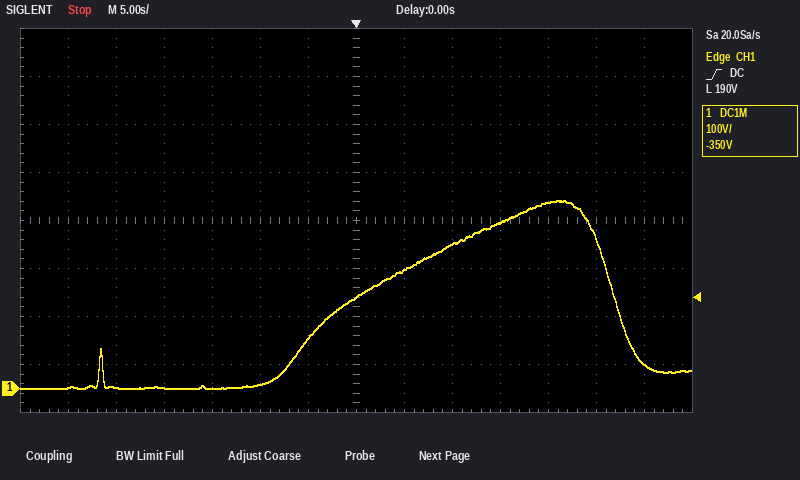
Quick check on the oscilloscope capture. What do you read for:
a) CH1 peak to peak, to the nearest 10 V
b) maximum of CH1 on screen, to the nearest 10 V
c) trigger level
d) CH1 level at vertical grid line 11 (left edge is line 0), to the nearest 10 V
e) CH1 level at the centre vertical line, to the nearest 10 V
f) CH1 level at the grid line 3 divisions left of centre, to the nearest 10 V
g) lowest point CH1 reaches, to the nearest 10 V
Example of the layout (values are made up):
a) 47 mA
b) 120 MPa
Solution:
a) 390 V
b) 390 V
c) 190 V
d) 390 V
e) 190 V
f) 0 V
g) 0 V
